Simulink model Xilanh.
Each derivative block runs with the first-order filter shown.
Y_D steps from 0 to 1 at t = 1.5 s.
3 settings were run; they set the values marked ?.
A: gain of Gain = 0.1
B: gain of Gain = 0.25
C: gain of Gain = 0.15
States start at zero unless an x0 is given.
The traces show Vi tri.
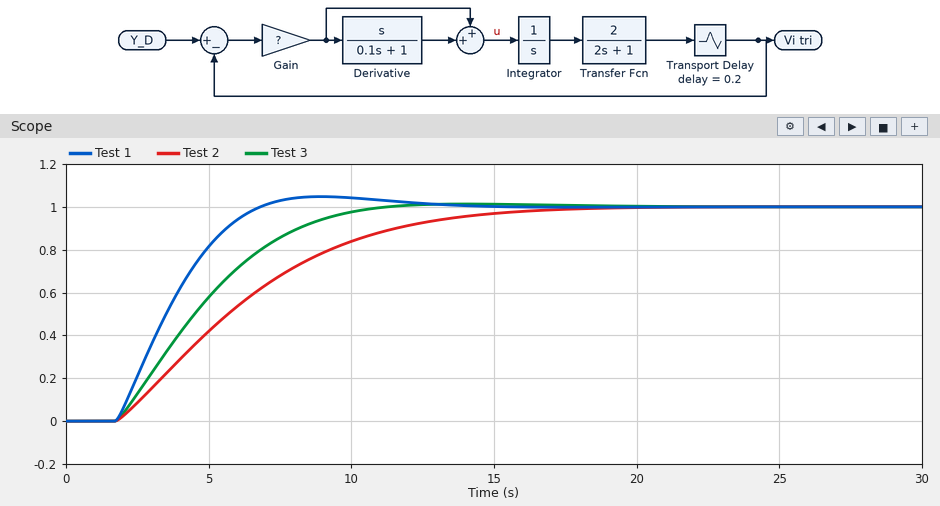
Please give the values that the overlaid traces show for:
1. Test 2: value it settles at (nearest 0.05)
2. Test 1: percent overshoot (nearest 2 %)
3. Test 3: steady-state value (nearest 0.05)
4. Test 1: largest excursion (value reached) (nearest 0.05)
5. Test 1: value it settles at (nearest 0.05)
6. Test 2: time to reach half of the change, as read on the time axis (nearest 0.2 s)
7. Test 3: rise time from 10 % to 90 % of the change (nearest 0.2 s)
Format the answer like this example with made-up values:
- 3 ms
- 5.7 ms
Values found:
- 1.00
- 4 %
- 1.00
- 1.05
- 1.00
- 5.6 s
- 5.8 s
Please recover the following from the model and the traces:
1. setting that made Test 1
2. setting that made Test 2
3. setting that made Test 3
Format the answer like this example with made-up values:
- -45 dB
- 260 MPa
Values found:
- B
- A
- C
